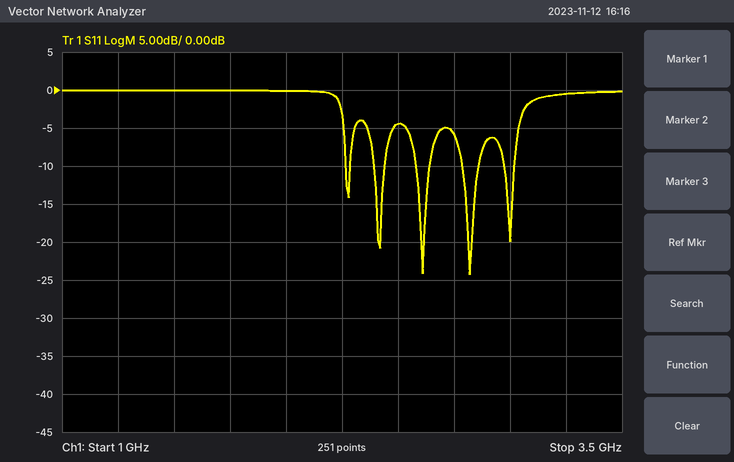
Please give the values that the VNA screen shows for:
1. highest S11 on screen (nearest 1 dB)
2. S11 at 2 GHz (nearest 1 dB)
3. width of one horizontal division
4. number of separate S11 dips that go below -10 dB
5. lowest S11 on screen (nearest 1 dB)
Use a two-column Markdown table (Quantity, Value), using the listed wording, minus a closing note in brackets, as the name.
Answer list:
| Quantity | Value |
|---|---|
| highest S11 on screen | 0 dB |
| S11 at 2 GHz | 0 dB |
| width of one horizontal division | 250 MHz |
| number of separate S11 dips that go below -10 dB | 5 |
| lowest S11 on screen | -24 dB |
